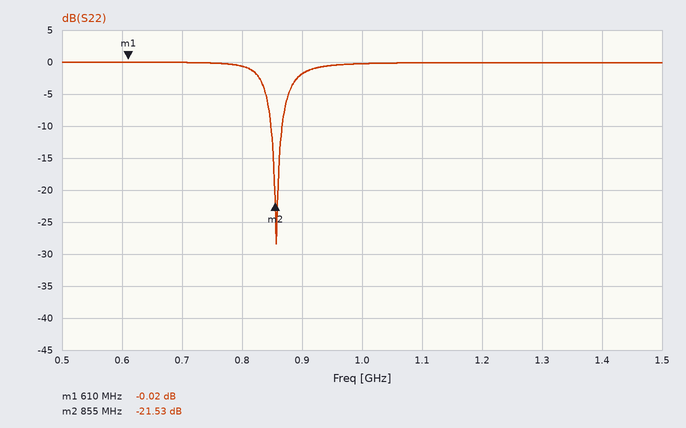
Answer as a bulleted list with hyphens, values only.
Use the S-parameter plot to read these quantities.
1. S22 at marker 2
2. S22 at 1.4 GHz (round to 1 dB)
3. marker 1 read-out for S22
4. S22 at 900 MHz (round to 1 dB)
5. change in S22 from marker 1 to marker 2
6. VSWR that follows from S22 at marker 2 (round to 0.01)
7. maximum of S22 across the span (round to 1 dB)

- -21.53 dB
- 0 dB
- -0.02 dB
- -2 dB
- -21.51 dB
- 1.18
- 0 dB
